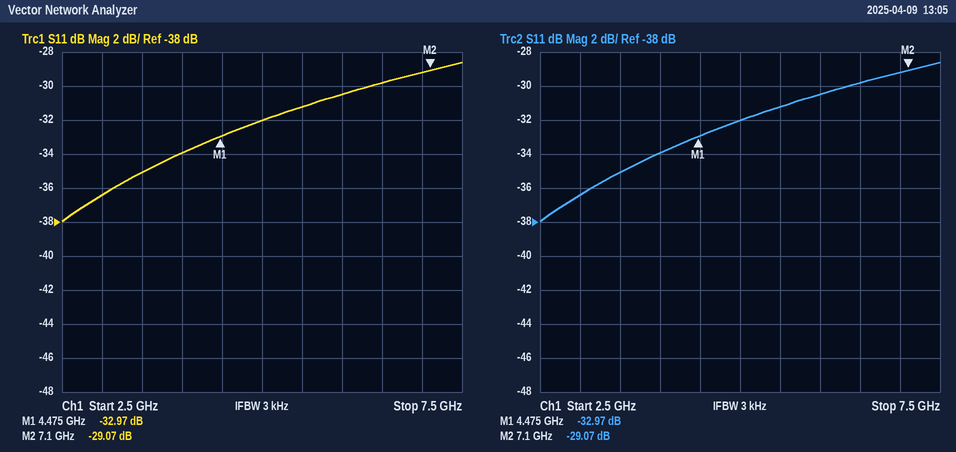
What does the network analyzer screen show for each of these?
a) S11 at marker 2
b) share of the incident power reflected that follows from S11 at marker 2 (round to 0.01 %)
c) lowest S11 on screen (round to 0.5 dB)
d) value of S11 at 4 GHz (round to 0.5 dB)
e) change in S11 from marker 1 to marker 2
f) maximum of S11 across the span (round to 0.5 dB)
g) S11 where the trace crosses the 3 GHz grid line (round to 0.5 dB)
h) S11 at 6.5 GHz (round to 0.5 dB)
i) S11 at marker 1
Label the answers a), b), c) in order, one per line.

a) -29.07 dB
b) 0.12 %
c) -38.0 dB
d) -34.0 dB
e) 3.90 dB
f) -28.5 dB
g) -36.5 dB
h) -30.0 dB
i) -32.97 dB
